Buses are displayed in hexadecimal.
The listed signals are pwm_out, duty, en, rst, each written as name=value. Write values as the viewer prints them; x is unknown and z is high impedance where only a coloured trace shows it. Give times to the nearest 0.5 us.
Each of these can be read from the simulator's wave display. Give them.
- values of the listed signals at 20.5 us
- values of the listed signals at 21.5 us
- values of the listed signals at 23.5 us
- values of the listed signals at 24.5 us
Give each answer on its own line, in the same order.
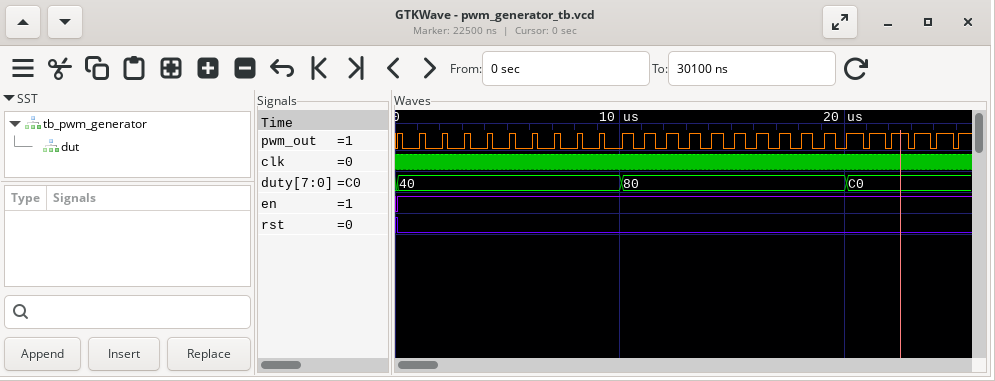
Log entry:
pwm_out=1, duty=C0, en=1, rst=0
pwm_out=1, duty=C0, en=1, rst=0
pwm_out=1, duty=C0, en=1, rst=0
pwm_out=1, duty=C0, en=1, rst=0
